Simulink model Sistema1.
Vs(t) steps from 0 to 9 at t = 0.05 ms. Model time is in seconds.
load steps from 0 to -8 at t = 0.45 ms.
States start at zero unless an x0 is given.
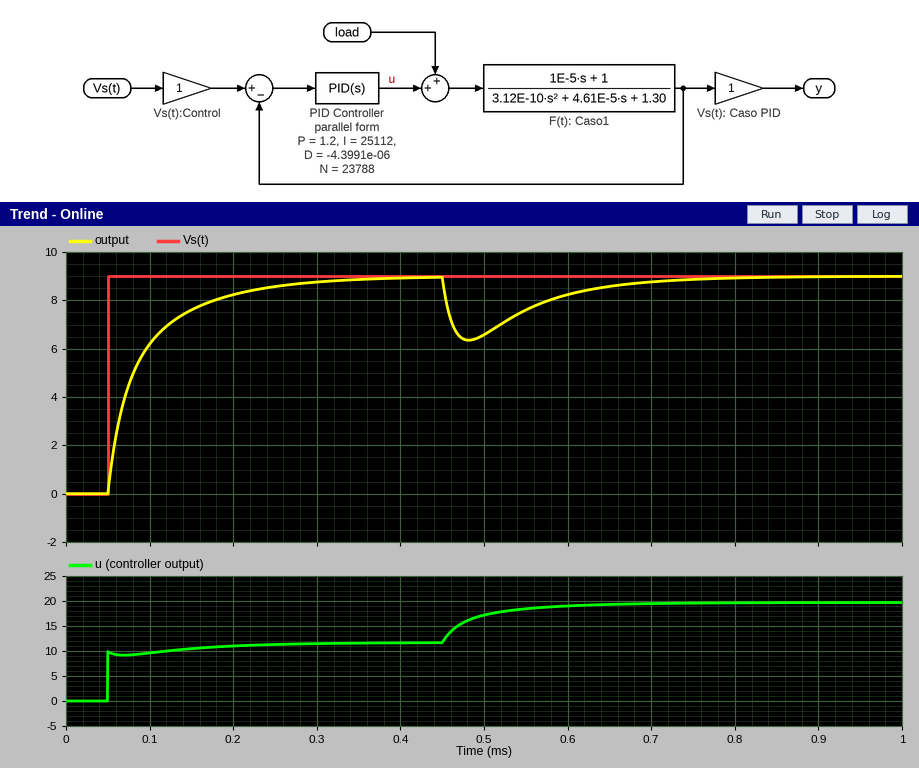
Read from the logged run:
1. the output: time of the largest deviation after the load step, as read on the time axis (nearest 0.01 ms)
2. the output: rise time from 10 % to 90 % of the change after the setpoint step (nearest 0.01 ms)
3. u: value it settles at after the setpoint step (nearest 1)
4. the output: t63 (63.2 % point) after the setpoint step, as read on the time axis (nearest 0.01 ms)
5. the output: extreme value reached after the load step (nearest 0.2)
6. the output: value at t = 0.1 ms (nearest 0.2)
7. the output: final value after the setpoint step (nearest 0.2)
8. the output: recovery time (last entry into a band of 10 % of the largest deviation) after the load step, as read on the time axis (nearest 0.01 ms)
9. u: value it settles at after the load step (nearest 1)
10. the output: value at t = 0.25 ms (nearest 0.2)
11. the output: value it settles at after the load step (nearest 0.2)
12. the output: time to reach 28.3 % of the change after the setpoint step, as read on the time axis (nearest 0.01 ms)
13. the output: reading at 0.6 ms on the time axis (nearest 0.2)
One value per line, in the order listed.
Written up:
0.48 ms
0.13 ms
12
0.09 ms
6.4
6.2
9.0
0.69 ms
20
8.6
9.0
0.06 ms
8.2
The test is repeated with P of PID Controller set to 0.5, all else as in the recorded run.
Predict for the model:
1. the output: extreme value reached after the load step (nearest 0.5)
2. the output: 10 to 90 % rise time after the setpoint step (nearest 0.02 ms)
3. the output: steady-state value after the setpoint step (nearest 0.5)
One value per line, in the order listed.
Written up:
5.5
0.10 ms
9.0
